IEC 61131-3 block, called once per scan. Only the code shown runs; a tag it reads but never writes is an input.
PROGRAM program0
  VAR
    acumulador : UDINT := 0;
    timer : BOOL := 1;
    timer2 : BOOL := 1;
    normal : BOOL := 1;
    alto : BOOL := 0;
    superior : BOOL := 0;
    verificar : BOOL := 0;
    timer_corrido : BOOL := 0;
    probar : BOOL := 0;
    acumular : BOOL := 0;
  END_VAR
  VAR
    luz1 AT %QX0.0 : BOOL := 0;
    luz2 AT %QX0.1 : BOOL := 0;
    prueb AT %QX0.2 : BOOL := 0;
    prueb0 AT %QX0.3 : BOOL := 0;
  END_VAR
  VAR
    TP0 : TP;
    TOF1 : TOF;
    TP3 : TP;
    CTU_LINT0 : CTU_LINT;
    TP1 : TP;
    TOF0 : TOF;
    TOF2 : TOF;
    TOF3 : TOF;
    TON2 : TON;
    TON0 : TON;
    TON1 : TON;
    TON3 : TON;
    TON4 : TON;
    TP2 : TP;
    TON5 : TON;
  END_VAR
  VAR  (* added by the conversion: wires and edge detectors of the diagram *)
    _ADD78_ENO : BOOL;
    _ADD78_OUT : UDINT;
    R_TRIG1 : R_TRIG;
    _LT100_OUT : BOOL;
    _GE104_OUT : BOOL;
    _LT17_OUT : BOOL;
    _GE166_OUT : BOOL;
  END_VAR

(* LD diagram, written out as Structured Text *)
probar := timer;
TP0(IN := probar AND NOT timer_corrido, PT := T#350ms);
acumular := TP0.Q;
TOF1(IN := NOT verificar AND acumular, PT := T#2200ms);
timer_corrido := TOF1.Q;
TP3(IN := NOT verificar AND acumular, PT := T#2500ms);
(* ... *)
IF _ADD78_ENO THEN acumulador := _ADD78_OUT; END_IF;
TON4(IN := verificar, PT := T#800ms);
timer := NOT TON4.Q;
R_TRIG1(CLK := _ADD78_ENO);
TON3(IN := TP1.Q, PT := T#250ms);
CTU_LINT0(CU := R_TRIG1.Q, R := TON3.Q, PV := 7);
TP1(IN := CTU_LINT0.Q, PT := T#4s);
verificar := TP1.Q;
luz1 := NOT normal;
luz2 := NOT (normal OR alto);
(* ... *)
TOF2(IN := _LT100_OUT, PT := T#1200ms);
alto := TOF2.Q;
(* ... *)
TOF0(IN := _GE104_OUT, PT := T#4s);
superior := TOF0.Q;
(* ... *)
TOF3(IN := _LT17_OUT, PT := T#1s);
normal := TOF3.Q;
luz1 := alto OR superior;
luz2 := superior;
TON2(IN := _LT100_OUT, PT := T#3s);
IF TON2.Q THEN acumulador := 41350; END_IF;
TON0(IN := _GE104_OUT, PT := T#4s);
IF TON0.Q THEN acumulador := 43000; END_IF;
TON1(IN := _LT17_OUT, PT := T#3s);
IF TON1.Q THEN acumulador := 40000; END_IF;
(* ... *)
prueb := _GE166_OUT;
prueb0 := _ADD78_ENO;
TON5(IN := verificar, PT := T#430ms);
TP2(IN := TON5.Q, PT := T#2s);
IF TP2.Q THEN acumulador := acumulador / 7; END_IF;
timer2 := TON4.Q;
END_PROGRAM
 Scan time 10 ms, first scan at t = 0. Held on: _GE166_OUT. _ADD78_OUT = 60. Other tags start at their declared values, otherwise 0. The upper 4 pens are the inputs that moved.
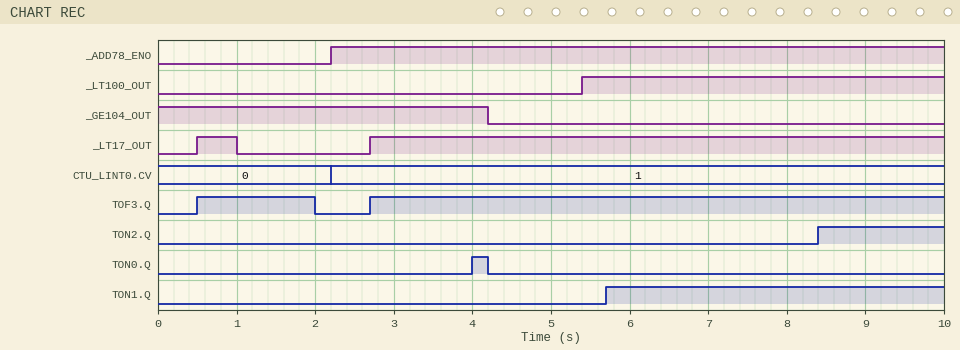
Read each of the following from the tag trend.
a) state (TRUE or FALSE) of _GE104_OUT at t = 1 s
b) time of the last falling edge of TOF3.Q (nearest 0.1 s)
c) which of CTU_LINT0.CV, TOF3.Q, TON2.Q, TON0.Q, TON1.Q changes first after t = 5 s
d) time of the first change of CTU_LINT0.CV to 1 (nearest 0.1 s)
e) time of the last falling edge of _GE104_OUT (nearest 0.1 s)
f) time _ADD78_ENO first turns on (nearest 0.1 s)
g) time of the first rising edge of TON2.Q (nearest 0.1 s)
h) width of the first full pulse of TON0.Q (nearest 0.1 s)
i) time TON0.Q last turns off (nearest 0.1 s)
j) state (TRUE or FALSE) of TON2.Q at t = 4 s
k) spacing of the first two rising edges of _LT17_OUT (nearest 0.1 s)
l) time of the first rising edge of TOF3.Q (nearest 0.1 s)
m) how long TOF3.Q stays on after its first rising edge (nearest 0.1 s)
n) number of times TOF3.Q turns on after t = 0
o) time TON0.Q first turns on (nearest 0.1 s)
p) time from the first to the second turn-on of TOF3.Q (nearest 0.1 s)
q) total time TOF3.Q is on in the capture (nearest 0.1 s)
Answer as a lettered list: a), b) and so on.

a) TRUE
b) 2.0 s
c) TON1.Q
d) 2.2 s
e) 4.2 s
f) 2.2 s
g) 8.4 s
h) 0.2 s
i) 4.2 s
j) FALSE
k) 2.2 s
l) 0.5 s
m) 1.5 s
n) 2
o) 4.0 s
p) 2.2 s
q) 8.8 s
